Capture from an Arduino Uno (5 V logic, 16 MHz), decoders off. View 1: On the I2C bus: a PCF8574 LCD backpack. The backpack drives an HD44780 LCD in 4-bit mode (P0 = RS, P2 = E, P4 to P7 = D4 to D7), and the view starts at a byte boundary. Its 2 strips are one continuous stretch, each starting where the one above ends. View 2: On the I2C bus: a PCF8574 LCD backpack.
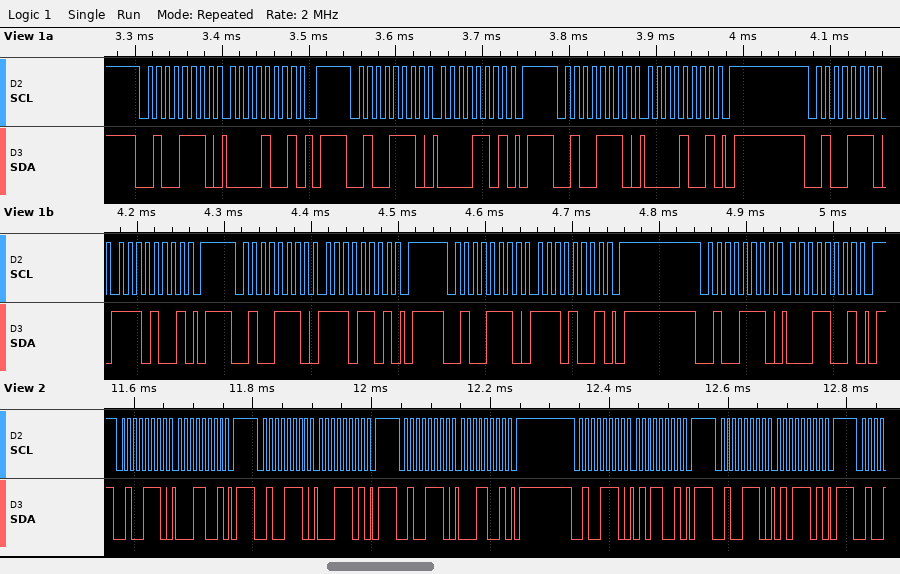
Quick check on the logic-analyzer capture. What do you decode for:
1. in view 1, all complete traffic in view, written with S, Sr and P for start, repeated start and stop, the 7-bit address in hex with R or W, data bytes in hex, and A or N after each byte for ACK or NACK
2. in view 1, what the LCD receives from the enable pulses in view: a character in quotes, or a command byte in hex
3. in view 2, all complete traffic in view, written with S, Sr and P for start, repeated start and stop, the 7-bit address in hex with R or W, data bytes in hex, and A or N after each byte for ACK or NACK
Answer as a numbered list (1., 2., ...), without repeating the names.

1. S 27W A 09 A P S 27W A 0D A P S 27W A 09 A P S 27W A E9 A P S 27W A ED A P S 27W A E9 A P S 27W A 19 A P
2. data 0x0E
3. S 27W A 19 A P S 27W A 1D A P S 27W A 19 A P S 27W A 59 A P S 27W A 5D A P
